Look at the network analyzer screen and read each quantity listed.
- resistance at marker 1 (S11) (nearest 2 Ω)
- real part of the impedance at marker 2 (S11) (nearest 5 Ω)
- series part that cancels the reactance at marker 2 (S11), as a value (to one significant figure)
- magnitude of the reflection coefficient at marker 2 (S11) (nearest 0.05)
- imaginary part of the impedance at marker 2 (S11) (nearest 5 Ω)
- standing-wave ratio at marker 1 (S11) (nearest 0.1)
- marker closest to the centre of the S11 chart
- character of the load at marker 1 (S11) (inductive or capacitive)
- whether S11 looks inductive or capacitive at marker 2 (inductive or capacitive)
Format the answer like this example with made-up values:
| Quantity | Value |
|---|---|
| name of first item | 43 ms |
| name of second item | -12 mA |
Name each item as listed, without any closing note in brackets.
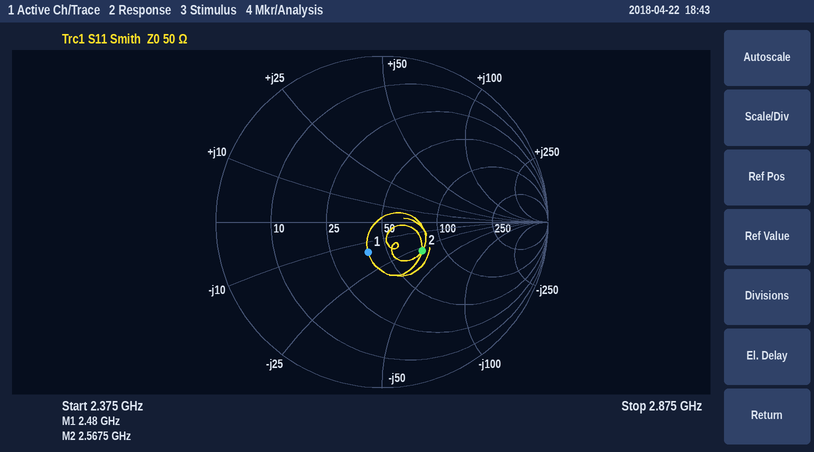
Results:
| Quantity | Value |
|---|---|
| resistance at marker 1 (S11) | 40 Ω |
| real part of the impedance at marker 2 (S11) | 75 Ω |
| series part that cancels the reactance at marker 2 (S11), as a value | 2 nH |
| magnitude of the reflection coefficient at marker 2 (S11) | 0.30 |
| imaginary part of the impedance at marker 2 (S11) | -30 Ω |
| standing-wave ratio at marker 1 (S11) | 1.5 |
| marker closest to the centre of the S11 chart | marker 1 |
| character of the load at marker 1 (S11) | capacitive |
| whether S11 looks inductive or capacitive at marker 2 | capacitive |
